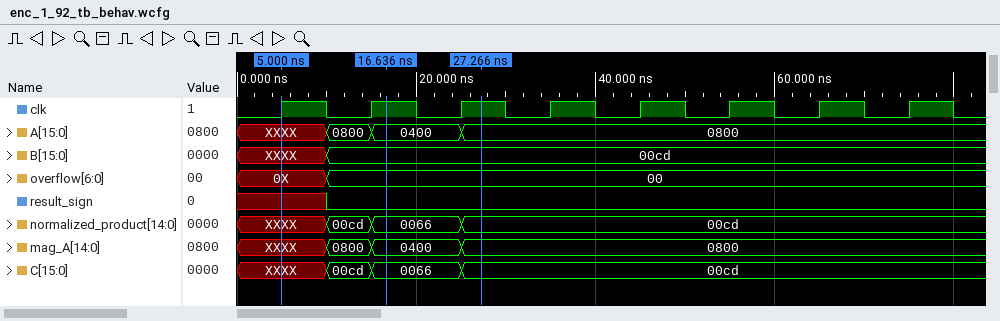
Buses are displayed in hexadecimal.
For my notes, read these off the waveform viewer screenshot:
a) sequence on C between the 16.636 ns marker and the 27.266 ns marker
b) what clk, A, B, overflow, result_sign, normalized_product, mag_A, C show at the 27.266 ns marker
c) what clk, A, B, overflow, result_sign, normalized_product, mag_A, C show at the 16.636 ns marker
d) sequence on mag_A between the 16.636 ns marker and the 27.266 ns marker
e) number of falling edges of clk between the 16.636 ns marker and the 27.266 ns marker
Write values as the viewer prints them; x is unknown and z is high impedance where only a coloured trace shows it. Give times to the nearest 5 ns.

0066, 00cd
clk=1, A=0800, B=00cd, overflow=00, result_sign=0, normalized_product=00cd, mag_A=0800, C=00cd
clk=1, A=0400, B=00cd, overflow=00, result_sign=0, normalized_product=0066, mag_A=0400, C=0066
0400, 0800
1
